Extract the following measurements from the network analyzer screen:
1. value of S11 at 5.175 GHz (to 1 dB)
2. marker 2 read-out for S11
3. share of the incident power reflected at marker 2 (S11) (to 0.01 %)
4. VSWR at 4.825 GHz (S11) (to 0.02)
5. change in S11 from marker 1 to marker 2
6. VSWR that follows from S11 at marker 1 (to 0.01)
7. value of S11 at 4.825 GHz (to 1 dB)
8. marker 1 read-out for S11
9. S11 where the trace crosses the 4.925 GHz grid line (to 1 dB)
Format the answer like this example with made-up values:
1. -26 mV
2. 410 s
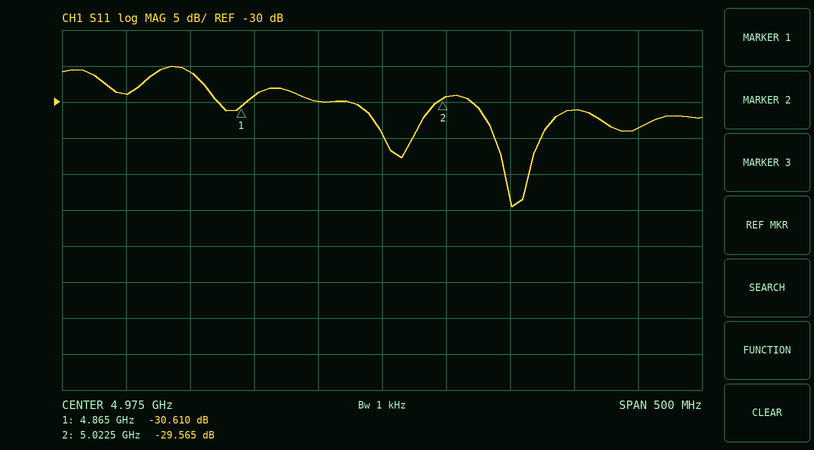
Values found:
1. -34 dB
2. -29.565 dB
3. 0.11 %
4. 1.10
5. 1.045 dB
6. 1.06
7. -26 dB
8. -30.610 dB
9. -30 dB
